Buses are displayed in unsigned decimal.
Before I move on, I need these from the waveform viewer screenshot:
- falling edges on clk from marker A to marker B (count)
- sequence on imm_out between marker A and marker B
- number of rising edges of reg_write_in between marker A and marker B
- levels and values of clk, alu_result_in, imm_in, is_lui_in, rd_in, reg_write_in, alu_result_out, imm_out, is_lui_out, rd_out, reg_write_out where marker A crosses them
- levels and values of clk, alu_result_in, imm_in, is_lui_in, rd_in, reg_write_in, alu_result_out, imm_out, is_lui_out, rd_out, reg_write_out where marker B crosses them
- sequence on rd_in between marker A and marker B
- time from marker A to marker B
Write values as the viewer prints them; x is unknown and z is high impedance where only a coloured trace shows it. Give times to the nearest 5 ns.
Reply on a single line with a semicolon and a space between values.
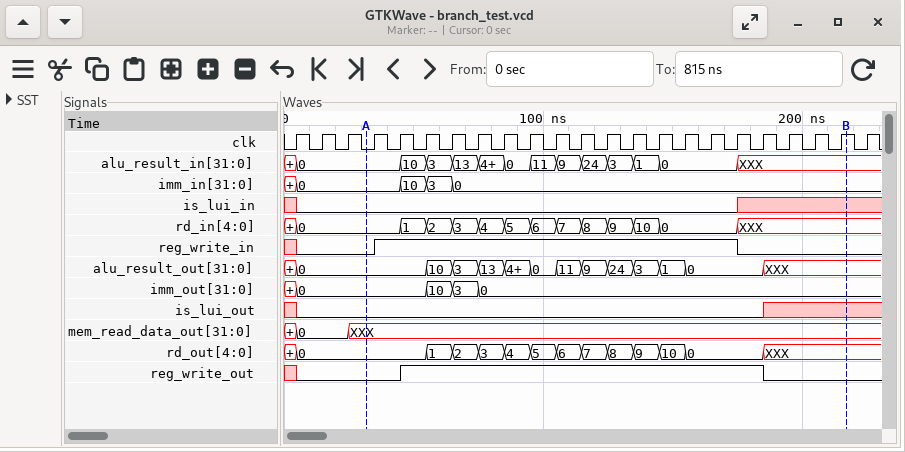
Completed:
18; 0, 10, 3, 0; 1; clk=0, alu_result_in=0, imm_in=0, is_lui_in=0, rd_in=0, reg_write_in=0, alu_result_out=0, imm_out=0, is_lui_out=0, rd_out=0, reg_write_out=0; clk=1, alu_result_in=XXX, imm_in=0, is_lui_in=x, rd_in=XXX, reg_write_in=0, alu_result_out=XXX, imm_out=0, is_lui_out=x, rd_out=XXX, reg_write_out=0; 0, 1, 2, 3, 4, 5, 6, 7, 8, 9, 10, 0, XXX; 185 ns
